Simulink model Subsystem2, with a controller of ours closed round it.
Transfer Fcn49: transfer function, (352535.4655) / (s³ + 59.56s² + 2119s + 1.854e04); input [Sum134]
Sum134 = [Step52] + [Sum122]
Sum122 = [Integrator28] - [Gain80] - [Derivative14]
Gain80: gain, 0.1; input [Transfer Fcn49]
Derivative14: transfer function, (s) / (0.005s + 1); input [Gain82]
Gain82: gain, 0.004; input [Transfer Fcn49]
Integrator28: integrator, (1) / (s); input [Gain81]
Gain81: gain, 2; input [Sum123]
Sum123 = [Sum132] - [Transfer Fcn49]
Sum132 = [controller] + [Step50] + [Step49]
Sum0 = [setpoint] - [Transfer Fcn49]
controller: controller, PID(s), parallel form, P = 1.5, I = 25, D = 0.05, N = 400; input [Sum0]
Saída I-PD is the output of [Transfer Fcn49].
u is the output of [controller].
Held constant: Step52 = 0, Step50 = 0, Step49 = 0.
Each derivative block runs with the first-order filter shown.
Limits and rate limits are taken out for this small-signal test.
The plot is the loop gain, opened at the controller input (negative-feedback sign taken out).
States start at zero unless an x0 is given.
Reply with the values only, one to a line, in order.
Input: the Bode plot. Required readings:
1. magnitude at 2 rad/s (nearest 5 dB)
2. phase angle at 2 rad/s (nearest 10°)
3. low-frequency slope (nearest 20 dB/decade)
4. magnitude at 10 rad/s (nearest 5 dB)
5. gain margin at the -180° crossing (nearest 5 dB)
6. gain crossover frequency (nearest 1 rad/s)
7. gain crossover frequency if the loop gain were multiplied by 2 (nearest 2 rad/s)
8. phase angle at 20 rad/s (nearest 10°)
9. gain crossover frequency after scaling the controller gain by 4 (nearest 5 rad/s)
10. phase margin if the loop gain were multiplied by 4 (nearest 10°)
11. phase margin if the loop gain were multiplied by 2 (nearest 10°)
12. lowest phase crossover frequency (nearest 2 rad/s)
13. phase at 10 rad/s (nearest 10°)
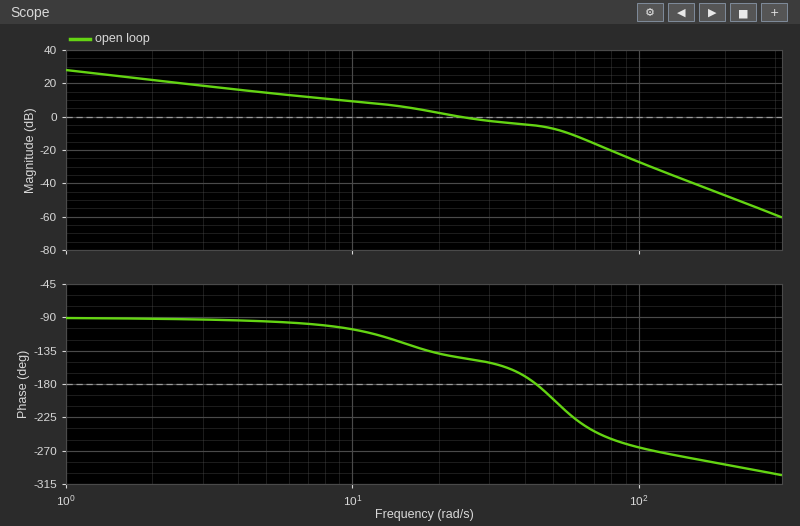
20 dB
-90°
-20 dB/decade
10 dB
5 dB
24 rad/s
46 rad/s
-140°
60 rad/s
-50°
-10°
44 rad/s
-110°
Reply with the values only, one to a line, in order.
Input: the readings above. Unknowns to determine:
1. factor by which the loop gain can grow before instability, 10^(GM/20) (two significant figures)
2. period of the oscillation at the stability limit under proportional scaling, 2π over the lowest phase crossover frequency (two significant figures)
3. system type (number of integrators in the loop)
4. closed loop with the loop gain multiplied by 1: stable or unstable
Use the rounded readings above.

1.8
0.14 s
1
stable
